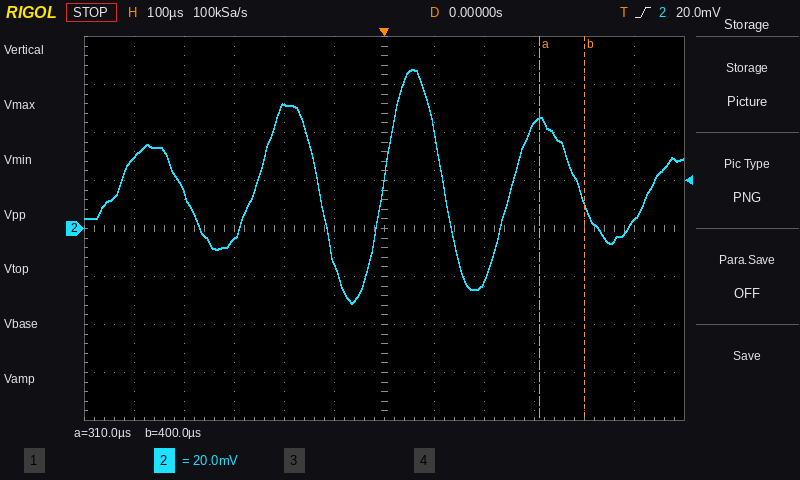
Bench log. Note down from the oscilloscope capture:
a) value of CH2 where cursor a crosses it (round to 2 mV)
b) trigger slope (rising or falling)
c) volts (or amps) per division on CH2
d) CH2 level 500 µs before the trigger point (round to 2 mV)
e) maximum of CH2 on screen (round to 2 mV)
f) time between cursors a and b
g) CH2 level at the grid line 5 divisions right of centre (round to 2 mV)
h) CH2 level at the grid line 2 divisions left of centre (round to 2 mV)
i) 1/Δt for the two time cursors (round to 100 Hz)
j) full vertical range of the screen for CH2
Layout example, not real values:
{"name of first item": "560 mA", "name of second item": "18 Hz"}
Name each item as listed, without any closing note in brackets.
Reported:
{"value of CH2 where cursor a crosses it": "46 mV", "trigger slope": "rising", "volts (or amps) per division on CH2": "20 mV", "CH2 level 500 µs before the trigger point": "30 mV", "maximum of CH2 on screen": "66 mV", "time between cursors a and b": "90 µs", "CH2 level at the grid line 5 divisions right of centre": "4 mV", "CH2 level at the grid line 2 divisions left of centre": "52 mV", "1/Δt for the two time cursors": "11.1 kHz", "full vertical range of the screen for CH2": "160 mV"}
